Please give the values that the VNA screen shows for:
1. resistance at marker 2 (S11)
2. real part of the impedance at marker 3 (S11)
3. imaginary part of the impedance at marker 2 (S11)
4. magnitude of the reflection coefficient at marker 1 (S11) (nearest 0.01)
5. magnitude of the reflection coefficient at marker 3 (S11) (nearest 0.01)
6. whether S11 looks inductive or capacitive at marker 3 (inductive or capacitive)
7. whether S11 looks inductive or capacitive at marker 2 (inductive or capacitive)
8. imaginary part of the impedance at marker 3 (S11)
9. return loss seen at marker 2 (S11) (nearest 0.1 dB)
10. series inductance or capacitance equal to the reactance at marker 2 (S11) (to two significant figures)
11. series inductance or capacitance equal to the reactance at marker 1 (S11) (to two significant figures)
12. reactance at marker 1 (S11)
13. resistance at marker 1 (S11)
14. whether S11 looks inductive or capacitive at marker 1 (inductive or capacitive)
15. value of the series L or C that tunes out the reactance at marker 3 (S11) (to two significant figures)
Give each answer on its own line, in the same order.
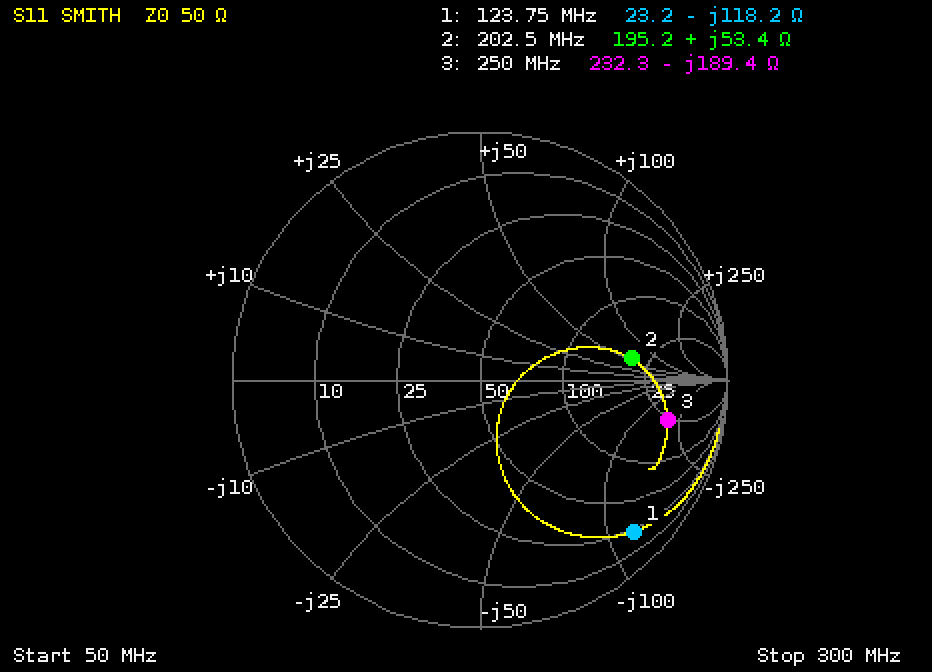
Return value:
195.2 Ω
232.3 Ω
+53.4 Ω
0.87
0.77
capacitive
inductive
-189.4 Ω
4.2 dB
42 nH
11 pF
-118.2 Ω
23.2 Ω
capacitive
120 nH
